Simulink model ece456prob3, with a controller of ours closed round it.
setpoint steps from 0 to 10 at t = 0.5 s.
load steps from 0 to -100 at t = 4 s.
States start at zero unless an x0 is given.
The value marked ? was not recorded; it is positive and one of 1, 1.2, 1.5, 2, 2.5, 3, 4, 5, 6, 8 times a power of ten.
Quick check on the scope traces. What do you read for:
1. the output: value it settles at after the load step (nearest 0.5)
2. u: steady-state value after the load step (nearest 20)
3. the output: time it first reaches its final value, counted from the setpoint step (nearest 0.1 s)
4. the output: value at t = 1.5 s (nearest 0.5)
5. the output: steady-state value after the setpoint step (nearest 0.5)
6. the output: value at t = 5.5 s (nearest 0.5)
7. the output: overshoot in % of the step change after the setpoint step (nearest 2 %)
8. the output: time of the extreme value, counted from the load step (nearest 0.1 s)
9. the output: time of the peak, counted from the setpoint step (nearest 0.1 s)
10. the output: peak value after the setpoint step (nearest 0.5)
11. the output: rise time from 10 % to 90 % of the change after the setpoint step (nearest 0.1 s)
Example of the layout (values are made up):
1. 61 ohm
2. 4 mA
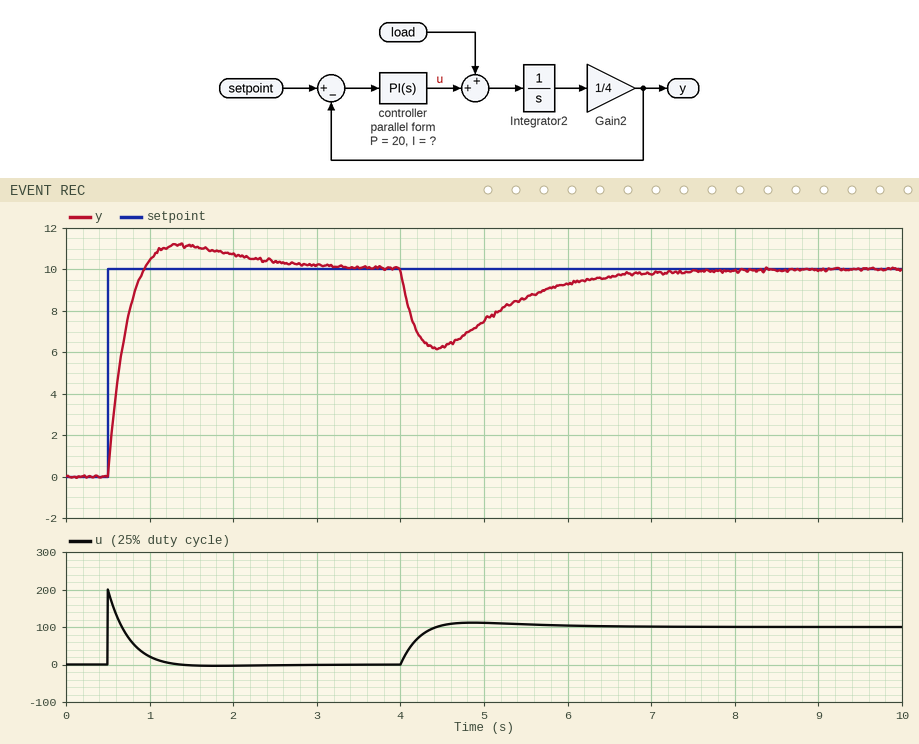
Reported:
1. 10.0
2. 100
3. 0.4 s
4. 11.0
5. 10.0
6. 8.5
7. 12 %
8. 0.4 s
9. 0.9 s
10. 11.0
11. 0.3 s
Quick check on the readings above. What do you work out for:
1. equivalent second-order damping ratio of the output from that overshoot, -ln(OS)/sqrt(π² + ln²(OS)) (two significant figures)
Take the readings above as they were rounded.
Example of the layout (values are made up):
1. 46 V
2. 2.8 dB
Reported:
1. 0.56
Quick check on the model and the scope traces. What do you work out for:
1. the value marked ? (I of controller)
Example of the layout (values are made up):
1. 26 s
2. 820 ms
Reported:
1. 20
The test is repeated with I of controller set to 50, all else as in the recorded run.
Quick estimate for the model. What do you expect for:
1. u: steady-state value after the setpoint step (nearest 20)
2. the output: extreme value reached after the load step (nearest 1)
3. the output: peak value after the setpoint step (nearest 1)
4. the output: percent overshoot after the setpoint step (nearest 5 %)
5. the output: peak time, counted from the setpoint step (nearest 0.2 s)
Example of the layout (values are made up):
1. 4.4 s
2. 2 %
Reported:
1. 0
2. 7
3. 12
4. 20 %
5. 0.6 s
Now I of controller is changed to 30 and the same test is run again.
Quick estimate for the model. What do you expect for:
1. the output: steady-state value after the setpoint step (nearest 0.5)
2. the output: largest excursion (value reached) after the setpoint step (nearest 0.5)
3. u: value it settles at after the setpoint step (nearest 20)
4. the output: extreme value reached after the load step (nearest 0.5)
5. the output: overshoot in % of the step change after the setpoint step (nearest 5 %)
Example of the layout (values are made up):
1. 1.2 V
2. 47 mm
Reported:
1. 10.0
2. 11.5
3. 0
4. 6.5
5. 15 %
